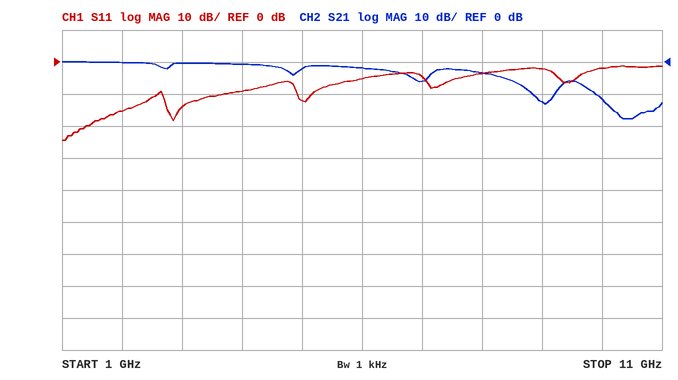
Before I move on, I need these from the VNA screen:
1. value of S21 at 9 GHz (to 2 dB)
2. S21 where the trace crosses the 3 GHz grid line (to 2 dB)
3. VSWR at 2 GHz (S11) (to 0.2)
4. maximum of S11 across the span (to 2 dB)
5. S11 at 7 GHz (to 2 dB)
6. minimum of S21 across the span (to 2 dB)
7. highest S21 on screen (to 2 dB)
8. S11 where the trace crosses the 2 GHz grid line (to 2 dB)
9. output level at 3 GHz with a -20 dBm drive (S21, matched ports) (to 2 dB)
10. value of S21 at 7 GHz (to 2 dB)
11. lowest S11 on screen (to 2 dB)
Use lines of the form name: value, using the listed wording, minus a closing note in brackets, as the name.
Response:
value of S21 at 9 GHz: -12 dB
S21 where the trace crosses the 3 GHz grid line: 0 dB
VSWR at 2 GHz (S11): 1.4
maximum of S11 across the span: -2 dB
S11 at 7 GHz: -4 dB
minimum of S21 across the span: -18 dB
highest S21 on screen: 0 dB
S11 where the trace crosses the 2 GHz grid line: -16 dB
output level at 3 GHz with a -20 dBm drive (S21, matched ports): -20 dBm
value of S21 at 7 GHz: -6 dB
lowest S11 on screen: -24 dB
